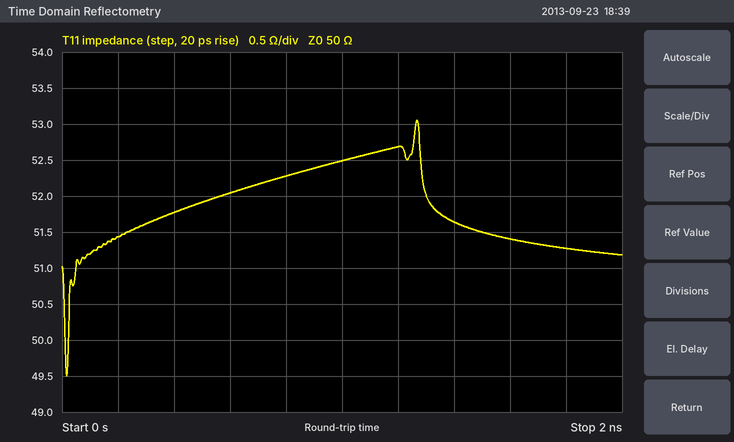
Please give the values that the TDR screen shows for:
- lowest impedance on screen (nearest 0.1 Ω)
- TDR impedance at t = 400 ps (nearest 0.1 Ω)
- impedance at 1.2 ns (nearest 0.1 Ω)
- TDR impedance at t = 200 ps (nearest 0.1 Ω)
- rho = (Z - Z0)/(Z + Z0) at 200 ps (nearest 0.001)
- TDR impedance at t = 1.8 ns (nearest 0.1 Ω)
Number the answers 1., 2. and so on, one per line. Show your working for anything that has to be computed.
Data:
1. 49.5 Ω
2. 51.8 Ω
3. 52.7 Ω
4. 51.4 Ω
5. (51.4 − 50)/(51.4 + 50) ≈ +0.014
6. 51.3 Ω
